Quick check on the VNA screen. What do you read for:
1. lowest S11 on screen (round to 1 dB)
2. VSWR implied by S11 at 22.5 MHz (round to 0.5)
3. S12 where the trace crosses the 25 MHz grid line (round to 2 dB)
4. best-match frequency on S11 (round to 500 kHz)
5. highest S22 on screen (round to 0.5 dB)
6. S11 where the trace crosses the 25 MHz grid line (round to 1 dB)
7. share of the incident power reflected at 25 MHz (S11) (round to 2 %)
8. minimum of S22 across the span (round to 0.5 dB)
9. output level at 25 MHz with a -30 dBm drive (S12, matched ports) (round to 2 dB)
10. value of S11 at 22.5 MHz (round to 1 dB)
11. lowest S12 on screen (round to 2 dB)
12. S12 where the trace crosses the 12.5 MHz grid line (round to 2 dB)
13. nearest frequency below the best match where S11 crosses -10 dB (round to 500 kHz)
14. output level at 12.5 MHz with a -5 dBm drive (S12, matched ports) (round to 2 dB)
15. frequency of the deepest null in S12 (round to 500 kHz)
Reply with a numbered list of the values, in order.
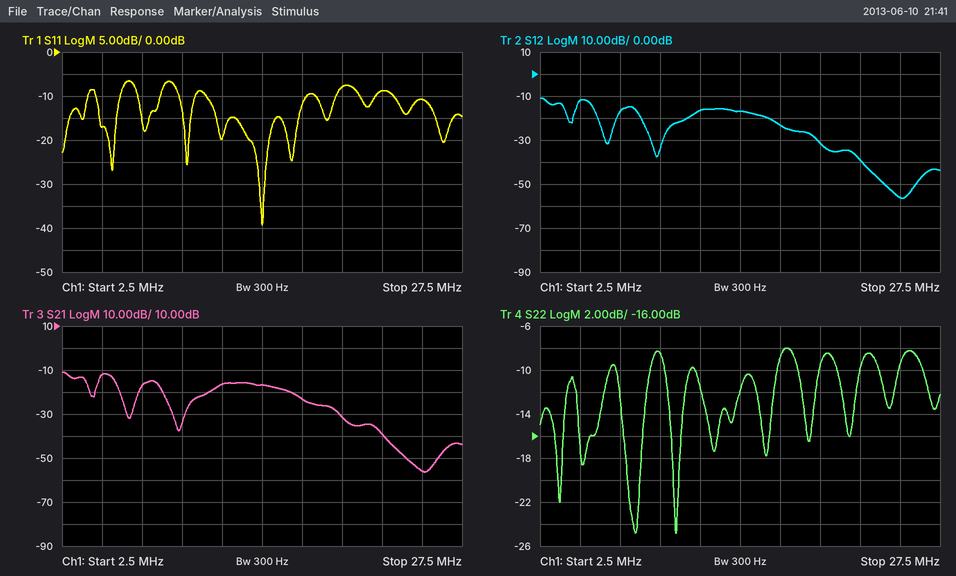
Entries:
1. -39 dB
2. 2.0
3. -56 dB
4. 15.0 MHz
5. -8.0 dB
6. -11 dB
7. 8 %
8. -25.0 dB
9. -86 dBm
10. -9 dB
11. -56 dB
12. -16 dB
13. 11.5 MHz
14. -22 dBm
15. 25.0 MHz
